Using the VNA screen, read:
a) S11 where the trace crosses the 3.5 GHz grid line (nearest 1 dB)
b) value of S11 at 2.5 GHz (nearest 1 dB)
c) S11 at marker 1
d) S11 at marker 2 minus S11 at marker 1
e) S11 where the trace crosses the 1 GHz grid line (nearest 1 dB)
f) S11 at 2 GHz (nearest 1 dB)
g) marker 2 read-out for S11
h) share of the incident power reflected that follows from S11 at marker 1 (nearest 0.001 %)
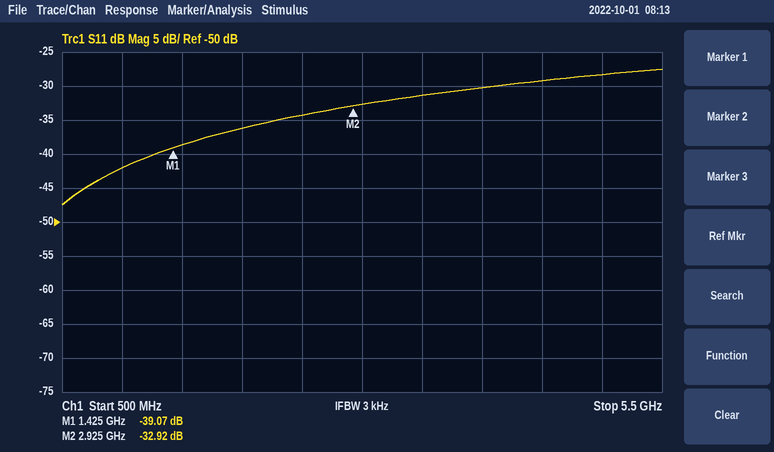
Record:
-31 dB
-34 dB
-39.07 dB
6.15 dB
-42 dB
-36 dB
-32.92 dB
0.012 %
